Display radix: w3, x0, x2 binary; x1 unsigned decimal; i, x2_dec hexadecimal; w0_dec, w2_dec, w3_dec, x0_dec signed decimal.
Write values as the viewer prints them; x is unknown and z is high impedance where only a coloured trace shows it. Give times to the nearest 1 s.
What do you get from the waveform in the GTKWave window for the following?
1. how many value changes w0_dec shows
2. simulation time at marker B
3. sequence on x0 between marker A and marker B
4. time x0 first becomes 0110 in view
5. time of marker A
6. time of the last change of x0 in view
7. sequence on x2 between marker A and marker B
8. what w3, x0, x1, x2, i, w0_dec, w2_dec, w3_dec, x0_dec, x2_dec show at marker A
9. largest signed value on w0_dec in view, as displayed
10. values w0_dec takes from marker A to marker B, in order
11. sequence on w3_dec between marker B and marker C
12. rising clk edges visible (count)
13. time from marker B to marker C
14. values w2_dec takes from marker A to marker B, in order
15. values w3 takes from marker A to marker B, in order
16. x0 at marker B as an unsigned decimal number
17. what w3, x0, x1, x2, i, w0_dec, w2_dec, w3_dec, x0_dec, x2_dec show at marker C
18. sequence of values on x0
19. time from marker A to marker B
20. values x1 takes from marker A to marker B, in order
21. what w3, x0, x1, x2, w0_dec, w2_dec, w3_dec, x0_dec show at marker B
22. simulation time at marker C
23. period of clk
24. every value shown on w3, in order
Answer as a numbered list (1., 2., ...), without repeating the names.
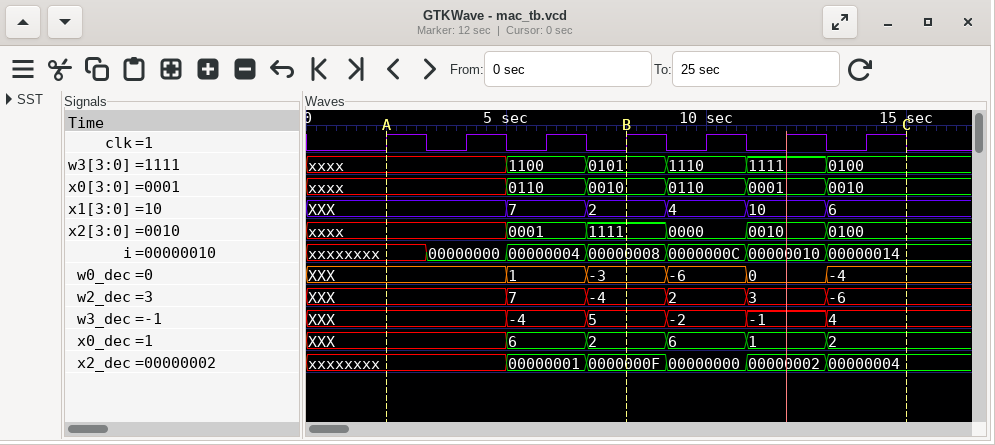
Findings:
1. 5
2. 8 s
3. xxxx, 0110, 0010
4. 5 s
5. 2 s
6. 13 s
7. xxxx, 0001, 1111
8. w3=xxxx, x0=xxxx, x1=XXX, x2=xxxx, i=xxxxxxxx, w0_dec=XXX, w2_dec=XXX, w3_dec=XXX, x0_dec=XXX, x2_dec=xxxxxxxx
9. 1
10. XXX, 1, -3
11. 5, -2, -1, 4
12. 7
13. 7 s
14. XXX, 7, -4
15. xxxx, 1100, 0101
16. 2
17. w3=0100, x0=0010, x1=6, x2=0100, i=00000014, w0_dec=-4, w2_dec=-6, w3_dec=4, x0_dec=2, x2_dec=00000004
18. xxxx, 0110, 0010, 0110, 0001, 0010
19. 6 s
20. XXX, 7, 2
21. w3=0101, x0=0010, x1=2, x2=1111, w0_dec=-3, w2_dec=-4, w3_dec=5, x0_dec=2
22. 15 s
23. 2 s
24. xxxx, 1100, 0101, 1110, 1111, 0100
